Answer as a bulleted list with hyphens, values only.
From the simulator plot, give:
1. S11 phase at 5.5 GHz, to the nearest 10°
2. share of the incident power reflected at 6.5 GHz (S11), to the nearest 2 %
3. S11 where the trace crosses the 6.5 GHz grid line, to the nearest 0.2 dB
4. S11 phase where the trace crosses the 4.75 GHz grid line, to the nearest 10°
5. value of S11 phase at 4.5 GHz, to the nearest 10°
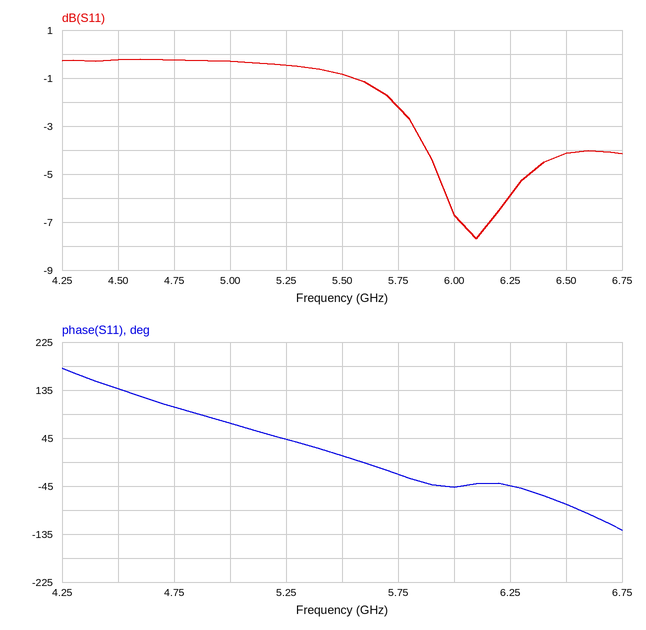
- 10°
- 38 %
- -4.2 dB
- 100°
- 140°
